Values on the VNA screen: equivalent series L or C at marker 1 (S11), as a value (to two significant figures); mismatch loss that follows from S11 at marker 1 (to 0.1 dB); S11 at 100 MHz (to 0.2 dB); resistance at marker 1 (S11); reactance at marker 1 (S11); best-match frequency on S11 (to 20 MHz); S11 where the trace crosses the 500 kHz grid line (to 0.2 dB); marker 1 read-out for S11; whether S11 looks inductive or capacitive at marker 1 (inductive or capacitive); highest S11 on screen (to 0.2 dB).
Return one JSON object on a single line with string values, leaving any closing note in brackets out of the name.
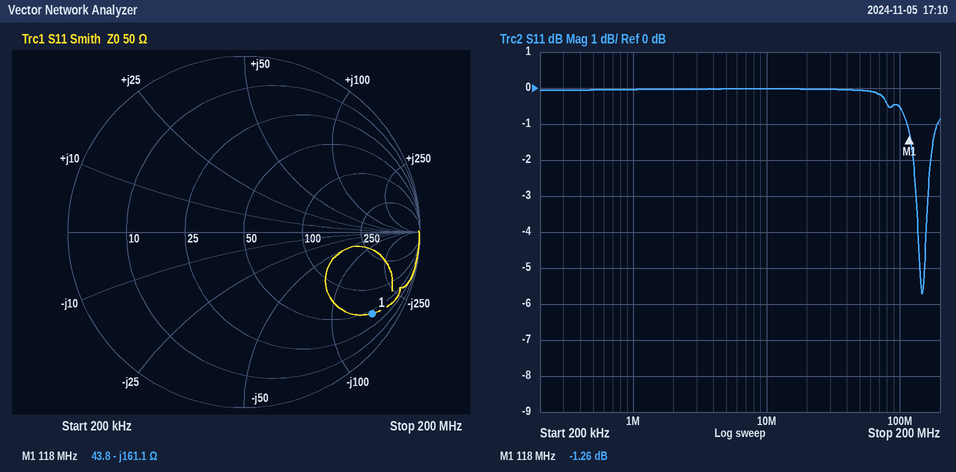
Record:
{"equivalent series L or C at marker 1 (S11), as a value": "8.4 pF", "mismatch loss that follows from S11 at marker 1": "6.0 dB", "S11 at 100 MHz": "-0.6 dB", "resistance at marker 1": "43.8 Ω", "reactance at marker 1": "-161.1 Ω", "best-match frequency on S11": "140 MHz", "S11 where the trace crosses the 500 kHz grid line": "0.0 dB", "marker 1 read-out for S11": "-1.26 dB", "whether S11 looks inductive or capacitive at marker 1": "capacitive", "highest S11 on screen": "0.0 dB"}
